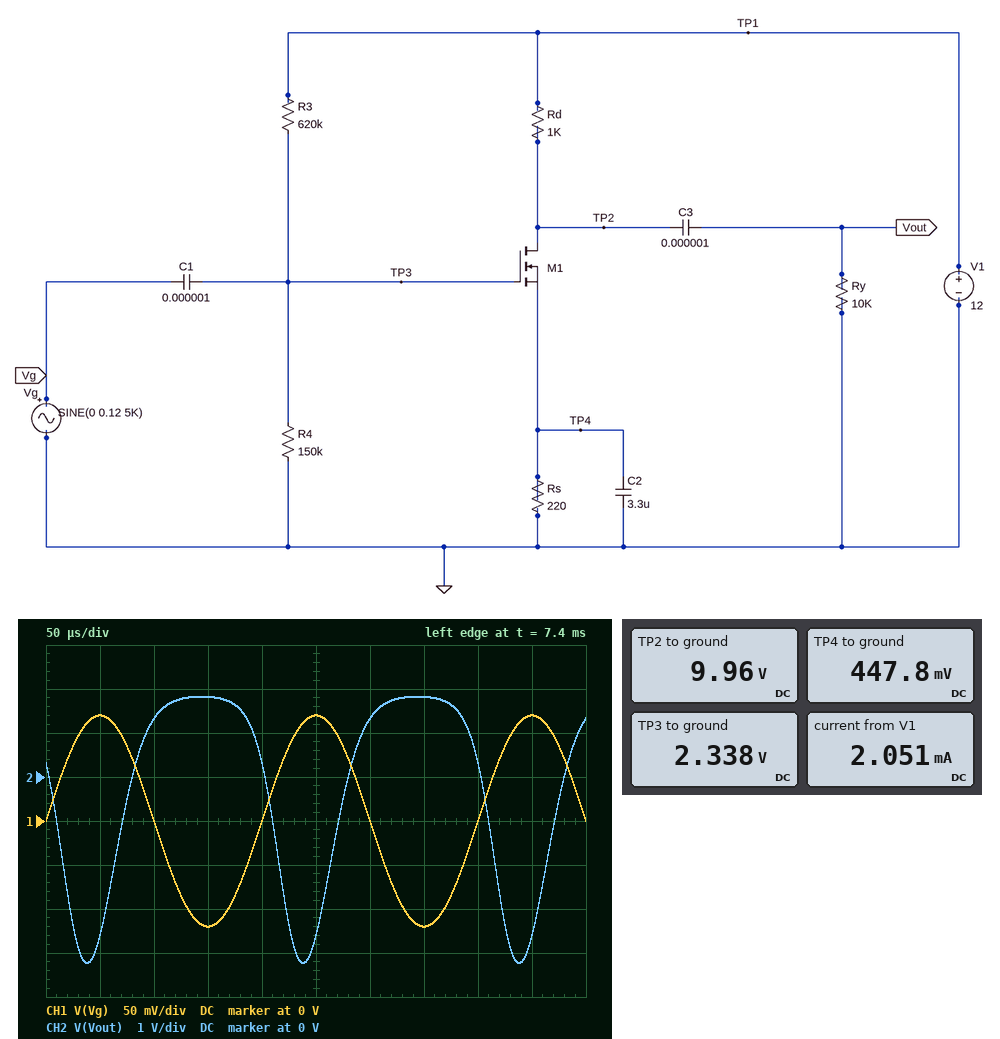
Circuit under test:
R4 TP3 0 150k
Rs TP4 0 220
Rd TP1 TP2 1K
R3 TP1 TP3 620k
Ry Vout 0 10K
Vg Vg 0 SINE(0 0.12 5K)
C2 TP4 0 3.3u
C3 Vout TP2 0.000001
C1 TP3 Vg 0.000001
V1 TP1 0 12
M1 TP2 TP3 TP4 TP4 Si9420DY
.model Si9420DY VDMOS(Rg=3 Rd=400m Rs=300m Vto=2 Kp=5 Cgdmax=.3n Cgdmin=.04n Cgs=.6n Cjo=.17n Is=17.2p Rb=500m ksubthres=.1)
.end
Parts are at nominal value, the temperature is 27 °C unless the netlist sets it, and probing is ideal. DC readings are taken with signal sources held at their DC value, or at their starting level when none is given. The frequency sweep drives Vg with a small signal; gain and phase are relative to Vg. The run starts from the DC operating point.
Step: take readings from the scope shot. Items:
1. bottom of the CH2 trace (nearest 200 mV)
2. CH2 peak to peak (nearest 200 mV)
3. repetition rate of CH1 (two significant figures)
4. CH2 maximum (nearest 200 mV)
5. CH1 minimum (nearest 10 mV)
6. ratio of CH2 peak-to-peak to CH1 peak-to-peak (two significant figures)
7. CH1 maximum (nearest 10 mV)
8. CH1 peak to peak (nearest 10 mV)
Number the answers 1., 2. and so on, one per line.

1. -4.2 V
2. 6.0 V
3. 5.0 kHz
4. 1.8 V
5. -120 mV
6. 25
7. 120 mV
8. 240 mV
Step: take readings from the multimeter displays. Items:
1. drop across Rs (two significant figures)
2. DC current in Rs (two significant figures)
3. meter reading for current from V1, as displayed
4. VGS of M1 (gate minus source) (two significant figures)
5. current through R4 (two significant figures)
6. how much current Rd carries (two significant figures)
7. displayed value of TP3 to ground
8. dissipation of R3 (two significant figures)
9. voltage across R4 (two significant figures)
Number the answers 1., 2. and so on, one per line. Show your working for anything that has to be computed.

1. 447.8 mV = 450 mV
2. (447.8 mV) / 220 Ω = 2.0 mA
3. 2.051 mA
4. 2.338 V - 447.8 mV = 1.9 V
5. (2.338 V) / 150 kΩ = 16 µA
6. (12 V - 9.96 V) / 1 kΩ = 2.0 mA
7. 2.338 V
8. (12 V - 2.338 V)^2 / 620 kΩ = 150 µW
9. 2.338 V = 2.3 V
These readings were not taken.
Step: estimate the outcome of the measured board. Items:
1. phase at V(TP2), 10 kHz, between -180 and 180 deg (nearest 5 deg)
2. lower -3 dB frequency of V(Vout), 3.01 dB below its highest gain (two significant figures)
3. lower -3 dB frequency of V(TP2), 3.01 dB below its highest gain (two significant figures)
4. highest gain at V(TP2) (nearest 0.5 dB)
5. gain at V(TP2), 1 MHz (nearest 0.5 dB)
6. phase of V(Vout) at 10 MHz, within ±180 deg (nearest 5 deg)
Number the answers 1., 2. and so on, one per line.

1. -170 deg
2. 1.9 kHz
3. 1.9 kHz
4. 30.0 dB
5. 28.5 dB
6. 85 deg
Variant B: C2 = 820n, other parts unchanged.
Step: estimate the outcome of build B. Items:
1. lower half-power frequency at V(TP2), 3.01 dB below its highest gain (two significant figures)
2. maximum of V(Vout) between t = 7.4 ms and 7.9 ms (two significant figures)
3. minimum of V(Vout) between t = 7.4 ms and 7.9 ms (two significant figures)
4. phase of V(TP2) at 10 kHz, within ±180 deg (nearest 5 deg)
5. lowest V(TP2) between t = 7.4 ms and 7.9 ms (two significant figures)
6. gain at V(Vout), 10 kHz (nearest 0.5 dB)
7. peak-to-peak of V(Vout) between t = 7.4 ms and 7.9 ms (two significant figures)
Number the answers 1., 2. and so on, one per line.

1. 7.5 kHz
2. 1.5 V
3. -2.4 V
4. -150 deg
5. 7.6 V
6. 28.0 dB
7. 3.9 V
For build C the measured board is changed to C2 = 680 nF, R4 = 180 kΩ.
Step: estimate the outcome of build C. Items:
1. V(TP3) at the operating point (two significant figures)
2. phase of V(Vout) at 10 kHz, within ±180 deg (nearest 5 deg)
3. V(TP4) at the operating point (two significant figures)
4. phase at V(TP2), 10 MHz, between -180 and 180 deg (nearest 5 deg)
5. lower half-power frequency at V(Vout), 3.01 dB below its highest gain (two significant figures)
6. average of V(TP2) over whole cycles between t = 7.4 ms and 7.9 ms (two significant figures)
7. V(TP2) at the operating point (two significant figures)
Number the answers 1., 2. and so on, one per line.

1. 2.7 V
2. -130 deg
3. 780 mV
4. 90 deg
5. 14 kHz
6. 8.4 V
7. 8.5 V
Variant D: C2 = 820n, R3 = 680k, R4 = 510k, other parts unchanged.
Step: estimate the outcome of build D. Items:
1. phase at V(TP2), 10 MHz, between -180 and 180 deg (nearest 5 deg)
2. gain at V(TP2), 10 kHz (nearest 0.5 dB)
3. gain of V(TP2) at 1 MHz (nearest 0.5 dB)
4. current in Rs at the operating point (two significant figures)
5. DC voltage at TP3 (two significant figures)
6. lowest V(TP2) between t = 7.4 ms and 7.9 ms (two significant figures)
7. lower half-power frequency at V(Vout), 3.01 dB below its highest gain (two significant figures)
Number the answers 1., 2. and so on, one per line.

1. 80 deg
2. -60.0 dB
3. -53.0 dB
4. 9.8 mA
5. 5.1 V
6. 2.2 V
7. 47 MHz
